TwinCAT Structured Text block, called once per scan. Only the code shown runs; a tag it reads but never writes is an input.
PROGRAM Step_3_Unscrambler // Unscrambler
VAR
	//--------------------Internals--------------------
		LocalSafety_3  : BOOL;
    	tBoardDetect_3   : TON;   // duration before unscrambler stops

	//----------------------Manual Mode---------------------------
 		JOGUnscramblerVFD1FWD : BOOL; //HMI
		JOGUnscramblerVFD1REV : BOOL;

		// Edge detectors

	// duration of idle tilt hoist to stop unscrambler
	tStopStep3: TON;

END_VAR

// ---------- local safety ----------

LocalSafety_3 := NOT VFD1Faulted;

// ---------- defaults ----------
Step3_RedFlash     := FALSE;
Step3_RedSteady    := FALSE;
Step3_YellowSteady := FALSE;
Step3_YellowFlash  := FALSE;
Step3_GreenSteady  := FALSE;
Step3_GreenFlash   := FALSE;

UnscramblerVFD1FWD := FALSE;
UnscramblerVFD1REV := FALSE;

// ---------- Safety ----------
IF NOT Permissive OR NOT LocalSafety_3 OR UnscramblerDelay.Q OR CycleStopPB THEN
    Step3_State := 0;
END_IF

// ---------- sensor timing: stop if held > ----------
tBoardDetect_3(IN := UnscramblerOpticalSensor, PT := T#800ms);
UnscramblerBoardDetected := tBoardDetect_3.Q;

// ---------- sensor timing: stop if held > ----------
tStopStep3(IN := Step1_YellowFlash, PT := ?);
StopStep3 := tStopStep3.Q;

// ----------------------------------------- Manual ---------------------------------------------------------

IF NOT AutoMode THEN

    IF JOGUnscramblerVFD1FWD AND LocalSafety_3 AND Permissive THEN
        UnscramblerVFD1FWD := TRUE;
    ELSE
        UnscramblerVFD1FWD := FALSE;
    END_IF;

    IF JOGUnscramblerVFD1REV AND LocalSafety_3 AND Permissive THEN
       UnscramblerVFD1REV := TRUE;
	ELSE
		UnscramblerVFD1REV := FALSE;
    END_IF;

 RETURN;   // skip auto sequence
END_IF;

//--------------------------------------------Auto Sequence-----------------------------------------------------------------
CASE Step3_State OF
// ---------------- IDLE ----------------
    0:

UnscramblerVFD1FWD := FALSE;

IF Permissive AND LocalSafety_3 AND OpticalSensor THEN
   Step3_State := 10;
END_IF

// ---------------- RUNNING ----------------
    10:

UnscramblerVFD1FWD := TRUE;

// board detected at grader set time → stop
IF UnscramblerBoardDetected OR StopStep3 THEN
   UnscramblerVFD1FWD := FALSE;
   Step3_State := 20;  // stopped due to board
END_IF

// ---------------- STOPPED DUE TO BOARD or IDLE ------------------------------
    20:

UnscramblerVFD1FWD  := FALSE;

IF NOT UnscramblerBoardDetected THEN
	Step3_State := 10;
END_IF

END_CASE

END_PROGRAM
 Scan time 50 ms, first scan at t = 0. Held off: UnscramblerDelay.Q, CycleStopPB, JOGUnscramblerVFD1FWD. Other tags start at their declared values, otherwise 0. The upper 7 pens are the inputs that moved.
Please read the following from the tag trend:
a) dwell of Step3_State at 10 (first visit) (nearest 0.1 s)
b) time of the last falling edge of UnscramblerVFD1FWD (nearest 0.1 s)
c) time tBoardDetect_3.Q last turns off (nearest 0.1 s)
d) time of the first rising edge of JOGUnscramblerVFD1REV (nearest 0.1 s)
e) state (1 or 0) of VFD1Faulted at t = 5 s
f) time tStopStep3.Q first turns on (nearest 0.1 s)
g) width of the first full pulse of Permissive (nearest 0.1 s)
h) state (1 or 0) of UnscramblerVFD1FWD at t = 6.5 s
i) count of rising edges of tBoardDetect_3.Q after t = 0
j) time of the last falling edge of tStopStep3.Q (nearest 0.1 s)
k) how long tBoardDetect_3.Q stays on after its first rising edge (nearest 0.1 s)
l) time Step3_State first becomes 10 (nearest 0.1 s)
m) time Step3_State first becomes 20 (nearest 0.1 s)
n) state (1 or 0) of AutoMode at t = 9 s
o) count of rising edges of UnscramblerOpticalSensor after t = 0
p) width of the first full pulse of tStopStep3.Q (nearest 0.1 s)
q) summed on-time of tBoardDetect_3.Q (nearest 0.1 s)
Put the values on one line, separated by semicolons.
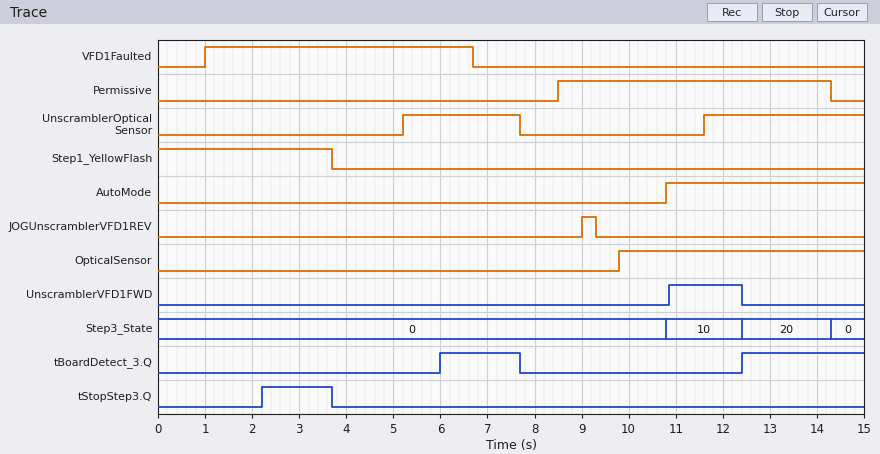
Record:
1.6 s; 12.4 s; 7.7 s; 9.0 s; 1; 2.2 s; 5.8 s; 0; 2; 3.7 s; 1.7 s; 10.8 s; 12.4 s; 0; 2; 1.5 s; 4.3 s
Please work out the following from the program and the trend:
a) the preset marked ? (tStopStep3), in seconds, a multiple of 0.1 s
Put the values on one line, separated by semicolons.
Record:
2.2 s
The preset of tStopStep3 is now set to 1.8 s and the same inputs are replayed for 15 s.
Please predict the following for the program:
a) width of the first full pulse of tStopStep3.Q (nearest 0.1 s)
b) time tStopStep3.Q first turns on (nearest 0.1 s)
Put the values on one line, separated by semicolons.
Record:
1.9 s; 1.8 s
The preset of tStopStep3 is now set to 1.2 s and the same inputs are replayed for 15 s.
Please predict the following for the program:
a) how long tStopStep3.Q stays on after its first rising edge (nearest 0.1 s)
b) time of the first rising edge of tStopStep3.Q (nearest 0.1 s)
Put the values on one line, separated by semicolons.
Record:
2.5 s; 1.2 s
